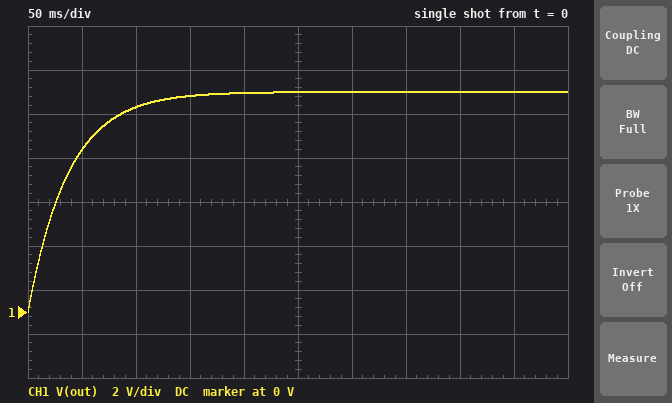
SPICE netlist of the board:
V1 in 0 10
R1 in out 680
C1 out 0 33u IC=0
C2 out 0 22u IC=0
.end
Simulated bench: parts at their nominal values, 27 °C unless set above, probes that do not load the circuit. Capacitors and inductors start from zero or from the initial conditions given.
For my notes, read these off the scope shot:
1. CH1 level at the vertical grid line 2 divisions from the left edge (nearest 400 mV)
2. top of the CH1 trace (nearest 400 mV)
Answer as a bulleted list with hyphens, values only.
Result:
- 9.2 V
- 10.0 V
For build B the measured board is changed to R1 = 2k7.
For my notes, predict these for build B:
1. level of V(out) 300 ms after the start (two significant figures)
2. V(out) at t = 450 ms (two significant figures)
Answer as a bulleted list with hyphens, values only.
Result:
- 8.7 V
- 9.5 V
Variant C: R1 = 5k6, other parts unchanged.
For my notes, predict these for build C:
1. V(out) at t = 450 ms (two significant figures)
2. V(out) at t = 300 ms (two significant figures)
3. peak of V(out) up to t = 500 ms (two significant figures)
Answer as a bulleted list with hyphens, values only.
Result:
- 7.7 V
- 6.2 V
- 8.0 V
